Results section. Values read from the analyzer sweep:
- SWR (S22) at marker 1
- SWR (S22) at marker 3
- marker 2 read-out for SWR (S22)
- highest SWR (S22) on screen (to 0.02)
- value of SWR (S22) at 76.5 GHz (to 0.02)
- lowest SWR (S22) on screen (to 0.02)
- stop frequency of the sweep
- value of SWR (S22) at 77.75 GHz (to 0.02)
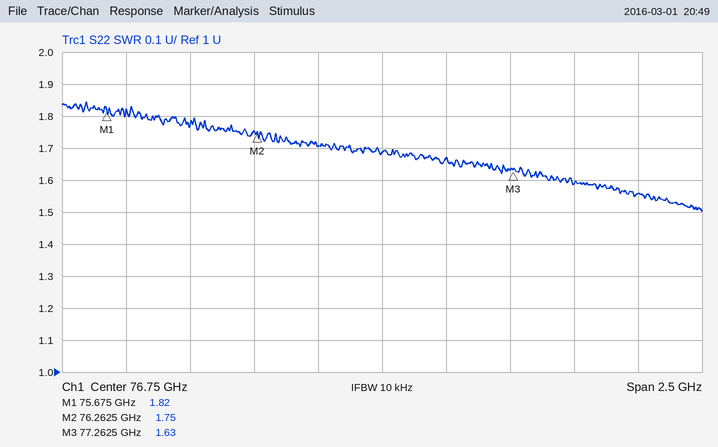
1.82
1.63
1.75
1.84
1.70
1.50
78 GHz
1.56
